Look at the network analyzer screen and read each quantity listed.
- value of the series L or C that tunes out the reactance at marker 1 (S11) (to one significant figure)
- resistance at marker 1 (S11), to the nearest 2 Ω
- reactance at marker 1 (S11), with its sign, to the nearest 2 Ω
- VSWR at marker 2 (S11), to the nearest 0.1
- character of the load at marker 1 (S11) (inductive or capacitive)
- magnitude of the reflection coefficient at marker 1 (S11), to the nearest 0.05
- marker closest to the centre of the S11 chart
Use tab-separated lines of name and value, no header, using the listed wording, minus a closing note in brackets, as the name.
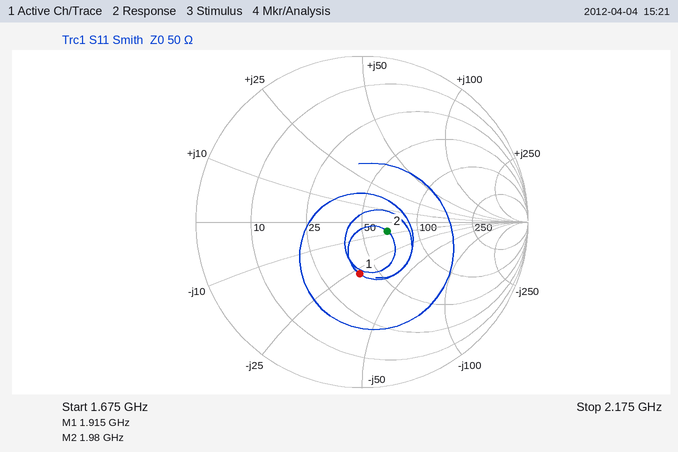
value of the series L or C that tunes out the reactance at marker 1 (S11)	2 nH
resistance at marker 1 (S11), to the nearest 2 Ω	40 Ω
reactance at marker 1 (S11), with its sign, to the nearest 2 Ω	-28 Ω
VSWR at marker 2 (S11), to the nearest 0.1	1.4
character of the load at marker 1 (S11)	capacitive
magnitude of the reflection coefficient at marker 1 (S11), to the nearest 0.05	0.30
marker closest to the centre of the S11 chart	marker 2
